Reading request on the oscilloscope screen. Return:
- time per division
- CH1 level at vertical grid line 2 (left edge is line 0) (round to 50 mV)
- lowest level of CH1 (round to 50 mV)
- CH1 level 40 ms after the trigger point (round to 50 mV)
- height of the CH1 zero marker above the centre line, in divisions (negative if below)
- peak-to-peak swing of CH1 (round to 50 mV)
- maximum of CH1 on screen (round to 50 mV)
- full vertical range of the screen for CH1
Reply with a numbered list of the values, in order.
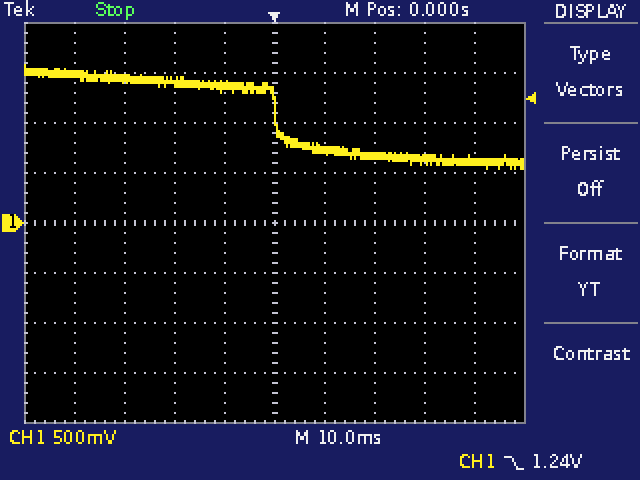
1. 10 ms
2. 1.45 V
3. 550 mV
4. 600 mV
5. 0.0 div
6. 1.05 V
7. 1.60 V
8. 4 V
